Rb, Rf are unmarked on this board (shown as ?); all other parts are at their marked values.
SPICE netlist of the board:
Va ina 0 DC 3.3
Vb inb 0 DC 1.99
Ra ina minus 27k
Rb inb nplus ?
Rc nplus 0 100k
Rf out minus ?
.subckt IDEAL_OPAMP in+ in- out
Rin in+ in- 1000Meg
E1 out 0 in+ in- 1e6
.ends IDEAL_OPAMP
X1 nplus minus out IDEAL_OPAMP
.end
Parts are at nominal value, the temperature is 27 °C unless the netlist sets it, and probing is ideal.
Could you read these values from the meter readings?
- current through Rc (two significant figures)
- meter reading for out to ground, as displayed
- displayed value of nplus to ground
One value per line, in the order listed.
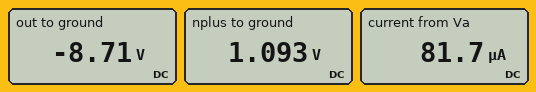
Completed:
11 µA
-8.71 V
1.093 V
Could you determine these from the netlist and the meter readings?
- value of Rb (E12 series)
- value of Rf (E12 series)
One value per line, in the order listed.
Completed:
82 kΩ
120 kΩ
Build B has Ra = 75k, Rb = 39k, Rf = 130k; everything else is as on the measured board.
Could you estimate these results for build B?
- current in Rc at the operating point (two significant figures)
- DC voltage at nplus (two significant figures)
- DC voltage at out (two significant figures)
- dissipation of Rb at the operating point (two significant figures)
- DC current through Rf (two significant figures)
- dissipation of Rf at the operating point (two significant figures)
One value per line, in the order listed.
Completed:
14 µA
1.4 V
-1.8 V
8.0 µW
25 µA
81 µW
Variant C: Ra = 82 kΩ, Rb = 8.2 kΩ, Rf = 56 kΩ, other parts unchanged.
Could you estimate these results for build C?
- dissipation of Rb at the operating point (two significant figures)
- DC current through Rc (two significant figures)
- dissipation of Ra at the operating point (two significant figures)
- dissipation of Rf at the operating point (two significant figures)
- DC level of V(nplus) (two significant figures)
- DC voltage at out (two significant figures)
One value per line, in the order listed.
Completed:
2.8 µW
18 µA
26 µW
18 µW
1.8 V
840 mV
